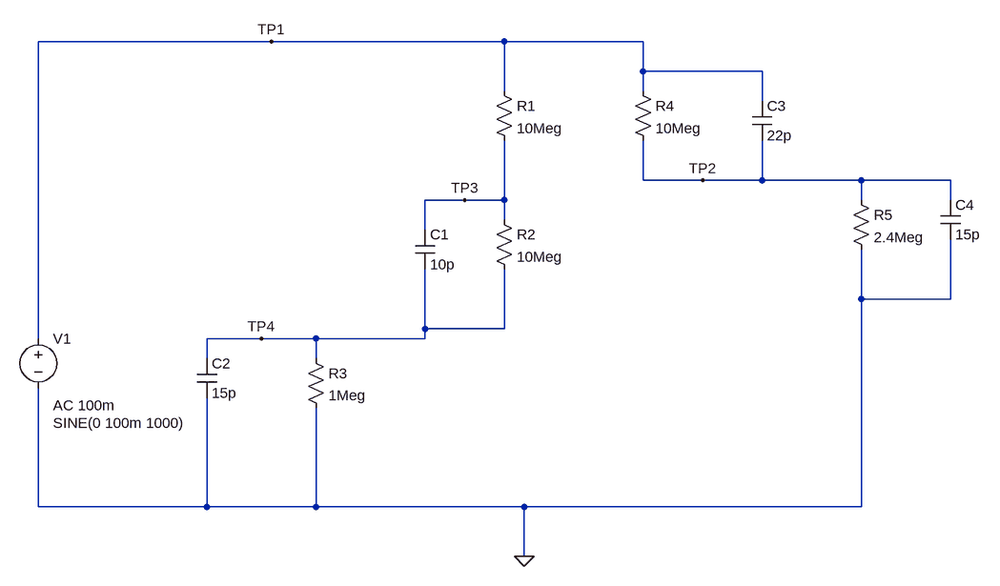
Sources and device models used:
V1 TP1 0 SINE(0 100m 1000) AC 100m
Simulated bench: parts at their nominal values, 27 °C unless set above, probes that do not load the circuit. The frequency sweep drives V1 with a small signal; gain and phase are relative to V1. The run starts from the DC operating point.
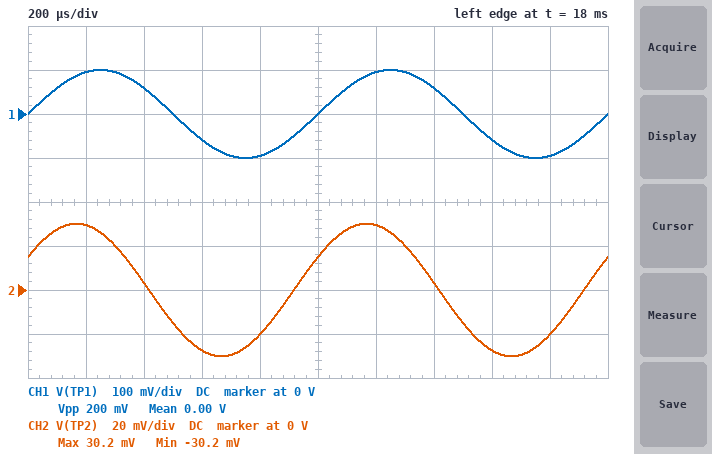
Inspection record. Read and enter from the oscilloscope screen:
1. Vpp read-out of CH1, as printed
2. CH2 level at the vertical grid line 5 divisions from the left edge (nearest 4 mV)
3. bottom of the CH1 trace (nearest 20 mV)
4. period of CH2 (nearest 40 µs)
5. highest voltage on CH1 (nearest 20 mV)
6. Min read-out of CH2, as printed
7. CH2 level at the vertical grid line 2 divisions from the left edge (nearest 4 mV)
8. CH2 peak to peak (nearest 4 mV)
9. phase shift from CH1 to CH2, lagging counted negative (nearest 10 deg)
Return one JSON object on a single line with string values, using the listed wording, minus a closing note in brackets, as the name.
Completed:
{"Vpp read-out of CH1, as printed": "200 mV", "CH2 level at the vertical grid line 5 divisions from the left edge": "16 mV", "bottom of the CH1 trace": "-100 mV", "period of CH2": "1.00 ms", "highest voltage on CH1": "100 mV", "Min read-out of CH2, as printed": "-30.2 mV", "CH2 level at the vertical grid line 2 divisions from the left edge": "4 mV", "CH2 peak to peak": "60 mV", "phase shift from CH1 to CH2, lagging counted negative": "30 deg"}
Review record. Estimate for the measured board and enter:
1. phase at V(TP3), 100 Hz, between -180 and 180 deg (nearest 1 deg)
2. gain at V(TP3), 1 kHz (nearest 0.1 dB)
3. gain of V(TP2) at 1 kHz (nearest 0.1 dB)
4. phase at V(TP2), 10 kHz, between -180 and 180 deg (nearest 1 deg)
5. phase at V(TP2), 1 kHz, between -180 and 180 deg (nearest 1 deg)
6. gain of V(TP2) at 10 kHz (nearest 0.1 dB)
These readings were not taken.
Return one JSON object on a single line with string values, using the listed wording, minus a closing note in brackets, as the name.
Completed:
{"phase at V(TP3), 100 Hz, between -180 and 180 deg": "-2 deg", "gain at V(TP3), 1 kHz": "-6.0 dB", "gain of V(TP2) at 1 kHz": "-10.4 dB", "phase at V(TP2), 10 kHz, between -180 and 180 deg": "8 deg", "phase at V(TP2), 1 kHz, between -180 and 180 deg": "30 deg", "gain of V(TP2) at 10 kHz": "-4.7 dB"}
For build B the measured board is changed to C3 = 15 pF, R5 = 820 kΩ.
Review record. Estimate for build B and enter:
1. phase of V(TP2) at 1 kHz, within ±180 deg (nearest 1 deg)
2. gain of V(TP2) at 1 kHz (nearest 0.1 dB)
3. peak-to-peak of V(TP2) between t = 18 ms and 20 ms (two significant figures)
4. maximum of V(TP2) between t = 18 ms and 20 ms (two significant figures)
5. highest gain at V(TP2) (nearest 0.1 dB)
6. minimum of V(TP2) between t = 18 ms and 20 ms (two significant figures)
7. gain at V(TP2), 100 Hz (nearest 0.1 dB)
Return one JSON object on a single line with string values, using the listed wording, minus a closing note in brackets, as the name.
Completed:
{"phase of V(TP2) at 1 kHz, within ±180 deg": "35 deg", "gain of V(TP2) at 1 kHz": "-19.7 dB", "peak-to-peak of V(TP2) between t = 18 ms and 20 ms": "21 mV", "maximum of V(TP2) between t = 18 ms and 20 ms": "10 mV", "highest gain at V(TP2)": "-6.0 dB", "minimum of V(TP2) between t = 18 ms and 20 ms": "-10 mV", "gain at V(TP2), 100 Hz": "-22.4 dB"}
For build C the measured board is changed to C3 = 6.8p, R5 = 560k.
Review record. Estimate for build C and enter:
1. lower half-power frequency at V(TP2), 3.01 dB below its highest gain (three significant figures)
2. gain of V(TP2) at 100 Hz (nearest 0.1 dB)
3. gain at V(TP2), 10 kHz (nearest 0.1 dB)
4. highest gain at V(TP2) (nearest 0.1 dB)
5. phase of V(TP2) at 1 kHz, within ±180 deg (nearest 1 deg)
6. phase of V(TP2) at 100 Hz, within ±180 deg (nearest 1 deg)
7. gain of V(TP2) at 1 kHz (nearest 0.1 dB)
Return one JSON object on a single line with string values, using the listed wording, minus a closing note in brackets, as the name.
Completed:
{"lower half-power frequency at V(TP2), 3.01 dB below its highest gain": "13.4 kHz", "gain of V(TP2) at 100 Hz": "-25.5 dB", "gain at V(TP2), 10 kHz": "-14.5 dB", "highest gain at V(TP2)": "-10.1 dB", "phase of V(TP2) at 1 kHz, within ±180 deg": "19 deg", "phase of V(TP2) at 100 Hz, within ±180 deg": "2 deg", "gain of V(TP2) at 1 kHz": "-24.8 dB"}
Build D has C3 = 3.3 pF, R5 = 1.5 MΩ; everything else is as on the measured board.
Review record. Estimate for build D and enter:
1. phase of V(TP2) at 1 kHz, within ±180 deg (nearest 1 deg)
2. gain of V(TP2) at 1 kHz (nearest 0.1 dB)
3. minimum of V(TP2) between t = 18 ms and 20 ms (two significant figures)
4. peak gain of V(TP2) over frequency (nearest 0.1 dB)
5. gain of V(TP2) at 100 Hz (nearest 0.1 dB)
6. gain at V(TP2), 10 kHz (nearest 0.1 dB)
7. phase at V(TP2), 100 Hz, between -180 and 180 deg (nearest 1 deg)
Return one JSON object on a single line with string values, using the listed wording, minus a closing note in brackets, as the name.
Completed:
{"phase of V(TP2) at 1 kHz, within ±180 deg": "3 deg", "gain of V(TP2) at 1 kHz": "-17.6 dB", "minimum of V(TP2) between t = 18 ms and 20 ms": "-13 mV", "peak gain of V(TP2) over frequency": "-14.9 dB", "gain of V(TP2) at 100 Hz": "-17.7 dB", "gain at V(TP2), 10 kHz": "-15.6 dB", "phase at V(TP2), 100 Hz, between -180 and 180 deg": "0 deg"}
